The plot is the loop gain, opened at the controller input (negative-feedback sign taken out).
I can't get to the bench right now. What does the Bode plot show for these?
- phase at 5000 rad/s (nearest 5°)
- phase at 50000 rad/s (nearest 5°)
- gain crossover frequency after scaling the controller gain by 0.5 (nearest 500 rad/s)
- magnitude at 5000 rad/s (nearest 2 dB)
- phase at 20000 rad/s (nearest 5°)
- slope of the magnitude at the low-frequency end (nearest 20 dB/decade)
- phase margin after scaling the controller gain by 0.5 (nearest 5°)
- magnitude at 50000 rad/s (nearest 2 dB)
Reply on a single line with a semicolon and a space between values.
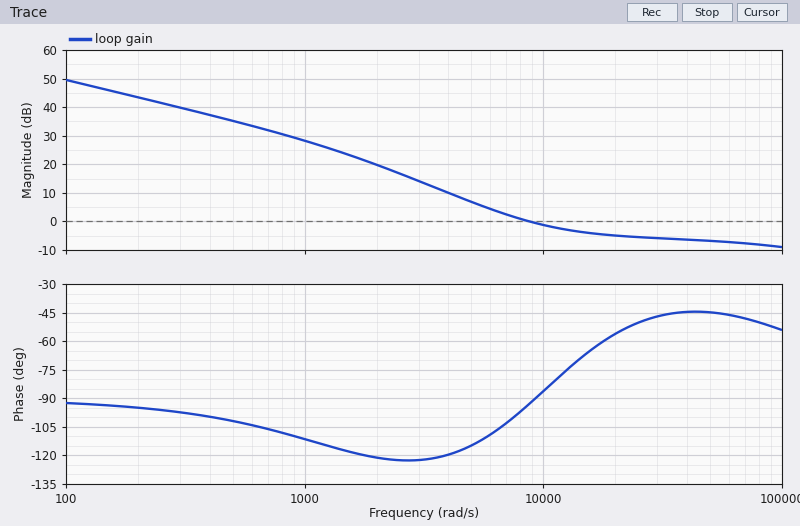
-115°; -45°; 5500 rad/s; 6 dB; -55°; -20 dB/decade; 65°; -6 dB
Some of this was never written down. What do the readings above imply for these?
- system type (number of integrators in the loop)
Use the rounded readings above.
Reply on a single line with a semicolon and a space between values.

1
